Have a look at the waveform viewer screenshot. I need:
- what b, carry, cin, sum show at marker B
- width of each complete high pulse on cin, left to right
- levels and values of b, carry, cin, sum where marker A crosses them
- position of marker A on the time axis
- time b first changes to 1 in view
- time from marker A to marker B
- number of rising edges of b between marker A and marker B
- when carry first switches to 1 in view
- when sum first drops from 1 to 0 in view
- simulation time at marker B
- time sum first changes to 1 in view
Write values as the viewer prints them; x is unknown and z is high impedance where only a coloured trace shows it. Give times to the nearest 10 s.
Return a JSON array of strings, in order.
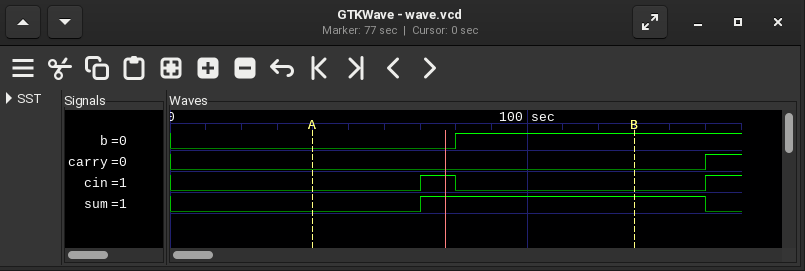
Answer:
["b=1, carry=0, cin=0, sum=1", "10 s", "b=0, carry=0, cin=0, sum=0", "40 s", "80 s", "90 s", "1", "150 s", "150 s", "130 s", "70 s"]
